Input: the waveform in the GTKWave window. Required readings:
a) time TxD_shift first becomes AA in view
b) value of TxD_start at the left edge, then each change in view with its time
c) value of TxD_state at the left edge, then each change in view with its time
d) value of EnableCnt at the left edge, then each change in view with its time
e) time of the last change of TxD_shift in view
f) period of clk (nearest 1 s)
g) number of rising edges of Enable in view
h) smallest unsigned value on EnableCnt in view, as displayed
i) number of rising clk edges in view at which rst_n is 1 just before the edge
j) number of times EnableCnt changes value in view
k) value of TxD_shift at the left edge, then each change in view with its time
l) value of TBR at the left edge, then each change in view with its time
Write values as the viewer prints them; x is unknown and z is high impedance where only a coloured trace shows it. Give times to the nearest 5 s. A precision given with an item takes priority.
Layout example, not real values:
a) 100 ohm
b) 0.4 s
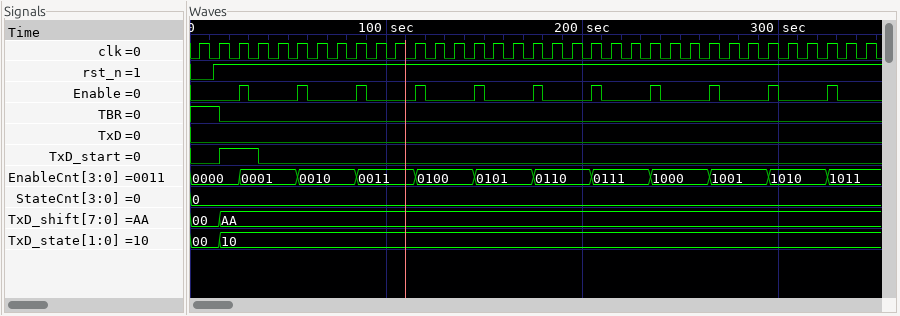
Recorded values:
a) 15 s
b) 0, 1 at 15 s, 0 at 35 s
c) 00, 10 at 15 s
d) 0000, 0001 at 25 s, 0010 at 55 s, 0011 at 85 s, 0100 at 115 s, 0101 at 145 s, 0110 at 175 s, 0111 at 205 s, 1000 at 235 s, 1001 at 265 s, 1010 at 295 s, 1011 at 325 s
e) 15 s
f) 10 s
g) 11
h) 0000
i) 34
j) 11
k) 00, AA at 15 s
l) 1, 0 at 15 s
